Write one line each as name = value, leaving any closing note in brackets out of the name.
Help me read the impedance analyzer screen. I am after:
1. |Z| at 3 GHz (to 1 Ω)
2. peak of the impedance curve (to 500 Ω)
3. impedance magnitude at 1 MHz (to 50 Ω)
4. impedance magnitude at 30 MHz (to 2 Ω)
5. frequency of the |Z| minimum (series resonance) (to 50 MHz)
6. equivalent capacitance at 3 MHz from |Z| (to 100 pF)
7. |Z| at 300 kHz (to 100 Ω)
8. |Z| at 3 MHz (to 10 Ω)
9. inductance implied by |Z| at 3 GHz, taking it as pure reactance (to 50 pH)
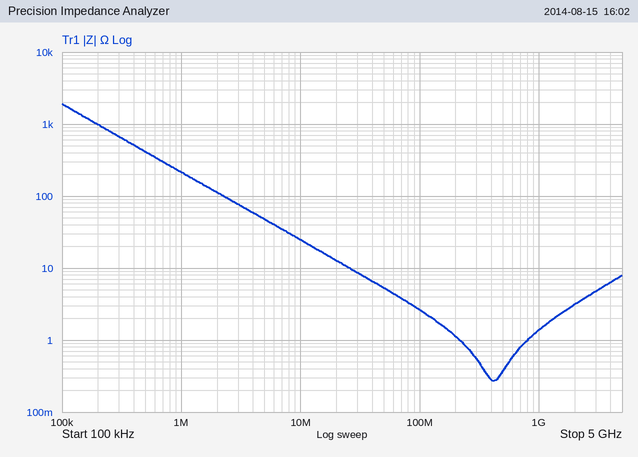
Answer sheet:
|Z| at 3 GHz = 5 Ω
peak of the impedance curve = 2.0 kΩ
impedance magnitude at 1 MHz = 200 Ω
impedance magnitude at 30 MHz = 8 Ω
frequency of the |Z| minimum (series resonance) = 400 MHz
equivalent capacitance at 3 MHz from |Z| = 700 pF
|Z| at 300 kHz = 700 Ω
|Z| at 3 MHz = 80 Ω
inductance implied by |Z| at 3 GHz, taking it as pure reactance = 250 pH
